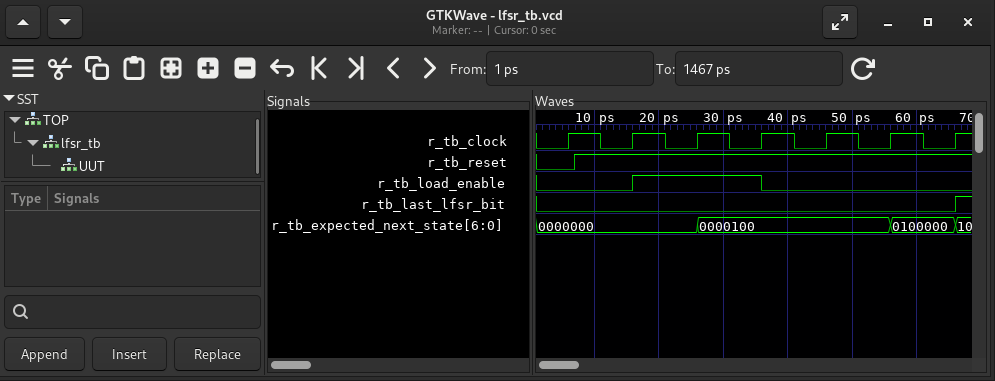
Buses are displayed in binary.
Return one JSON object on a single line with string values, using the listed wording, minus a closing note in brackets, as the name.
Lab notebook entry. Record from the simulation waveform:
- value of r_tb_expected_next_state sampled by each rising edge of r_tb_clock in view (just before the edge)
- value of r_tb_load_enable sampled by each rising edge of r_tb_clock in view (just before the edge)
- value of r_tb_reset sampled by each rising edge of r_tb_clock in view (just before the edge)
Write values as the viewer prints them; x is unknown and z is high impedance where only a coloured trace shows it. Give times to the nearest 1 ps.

{"value of r_tb_expected_next_state sampled by each rising edge of r_tb_clock in view": "0000000, 0000000, 0000000, 0000100, 0000100, 0000100, 0100000", "value of r_tb_load_enable sampled by each rising edge of r_tb_clock in view": "0 0 1 1 0 0 0", "value of r_tb_reset sampled by each rising edge of r_tb_clock in view": "0 1 1 1 1 1 1"}
